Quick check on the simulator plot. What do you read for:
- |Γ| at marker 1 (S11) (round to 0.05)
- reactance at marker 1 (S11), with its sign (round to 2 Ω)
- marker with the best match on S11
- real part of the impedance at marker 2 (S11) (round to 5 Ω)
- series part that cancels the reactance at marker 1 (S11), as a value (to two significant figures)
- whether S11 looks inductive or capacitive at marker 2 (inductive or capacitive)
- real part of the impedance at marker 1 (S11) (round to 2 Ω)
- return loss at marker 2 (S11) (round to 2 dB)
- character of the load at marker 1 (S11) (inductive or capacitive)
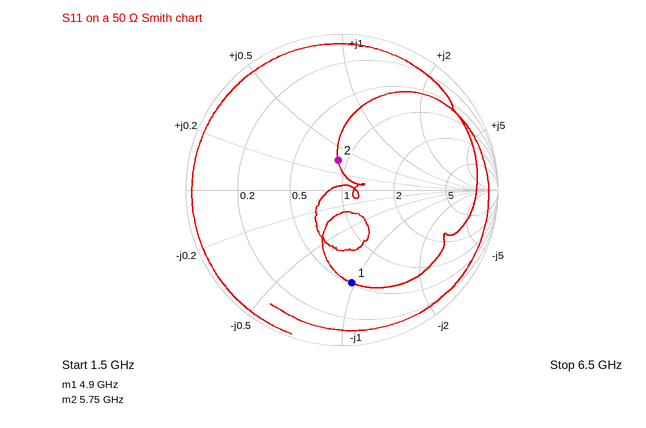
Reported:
0.60
-48 Ω
marker 2
45 Ω
1.6 nH
inductive
26 Ω
14 dB
capacitive
